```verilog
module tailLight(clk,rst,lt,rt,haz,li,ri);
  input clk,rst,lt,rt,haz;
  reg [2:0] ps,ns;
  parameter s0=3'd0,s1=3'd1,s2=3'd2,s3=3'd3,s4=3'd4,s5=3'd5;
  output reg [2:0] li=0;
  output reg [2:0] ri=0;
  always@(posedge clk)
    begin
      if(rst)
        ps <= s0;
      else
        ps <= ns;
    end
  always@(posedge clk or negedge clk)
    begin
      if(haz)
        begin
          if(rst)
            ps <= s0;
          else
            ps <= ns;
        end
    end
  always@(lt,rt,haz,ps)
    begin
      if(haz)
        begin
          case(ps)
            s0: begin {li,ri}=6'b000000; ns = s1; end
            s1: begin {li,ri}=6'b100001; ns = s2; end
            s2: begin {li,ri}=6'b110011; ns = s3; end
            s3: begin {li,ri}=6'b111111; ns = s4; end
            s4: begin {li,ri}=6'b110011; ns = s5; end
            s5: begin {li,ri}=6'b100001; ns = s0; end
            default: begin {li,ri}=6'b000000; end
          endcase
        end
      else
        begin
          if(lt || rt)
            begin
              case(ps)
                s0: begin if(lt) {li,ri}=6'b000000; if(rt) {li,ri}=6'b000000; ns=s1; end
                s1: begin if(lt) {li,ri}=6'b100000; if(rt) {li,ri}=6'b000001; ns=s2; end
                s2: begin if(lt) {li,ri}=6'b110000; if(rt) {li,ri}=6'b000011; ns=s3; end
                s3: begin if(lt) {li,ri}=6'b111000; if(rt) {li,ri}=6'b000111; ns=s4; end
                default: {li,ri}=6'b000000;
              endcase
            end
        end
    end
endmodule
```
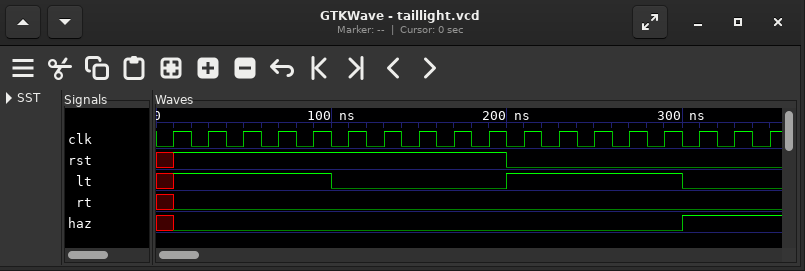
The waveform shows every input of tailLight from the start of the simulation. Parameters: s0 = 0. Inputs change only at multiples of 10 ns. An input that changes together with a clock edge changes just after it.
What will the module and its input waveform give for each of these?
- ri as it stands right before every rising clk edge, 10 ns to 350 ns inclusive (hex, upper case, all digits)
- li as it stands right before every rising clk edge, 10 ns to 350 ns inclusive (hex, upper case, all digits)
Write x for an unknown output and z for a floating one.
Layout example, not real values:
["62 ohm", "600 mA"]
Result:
["0, 0, 0, 0, 0, 0, 0, 0, 0, 0, 0, 0, 0, 0, 0, 3, 0, 3", "0, 0, 0, 0, 0, 0, 0, 0, 0, 0, 0, 4, 6, 7, 0, 6, 0, 6"]
